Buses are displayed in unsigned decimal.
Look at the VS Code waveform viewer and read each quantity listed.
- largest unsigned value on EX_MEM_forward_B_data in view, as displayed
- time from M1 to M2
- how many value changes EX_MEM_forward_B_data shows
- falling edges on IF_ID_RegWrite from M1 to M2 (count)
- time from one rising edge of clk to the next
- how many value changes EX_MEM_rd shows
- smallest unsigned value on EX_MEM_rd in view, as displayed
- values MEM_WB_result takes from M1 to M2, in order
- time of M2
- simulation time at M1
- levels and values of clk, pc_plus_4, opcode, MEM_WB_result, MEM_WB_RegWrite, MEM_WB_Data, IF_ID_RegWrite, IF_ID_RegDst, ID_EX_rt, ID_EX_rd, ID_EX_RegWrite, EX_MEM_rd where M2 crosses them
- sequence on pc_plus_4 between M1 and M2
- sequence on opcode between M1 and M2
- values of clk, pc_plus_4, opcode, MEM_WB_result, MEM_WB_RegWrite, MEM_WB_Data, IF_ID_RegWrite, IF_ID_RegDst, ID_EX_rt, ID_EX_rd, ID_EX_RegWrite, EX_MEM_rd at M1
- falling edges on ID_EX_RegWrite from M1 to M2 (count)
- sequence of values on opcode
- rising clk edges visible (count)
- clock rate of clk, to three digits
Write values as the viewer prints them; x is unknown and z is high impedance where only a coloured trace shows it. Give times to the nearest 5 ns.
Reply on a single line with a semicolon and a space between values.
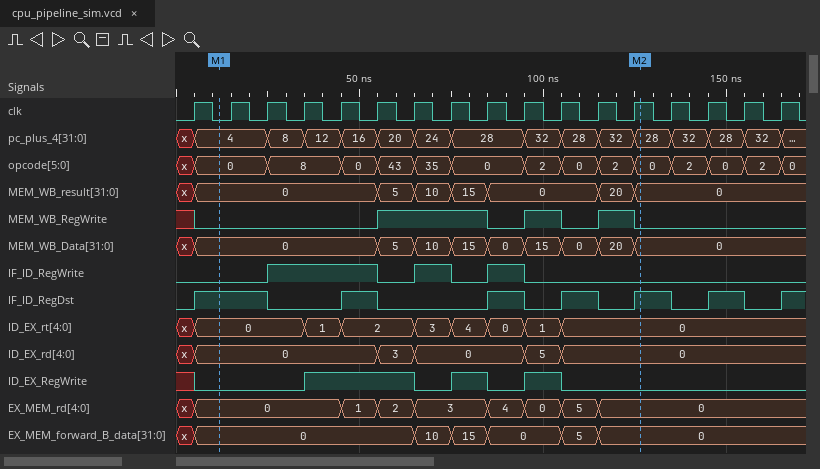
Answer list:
15; 115 ns; 6; 3; 10 ns; 8; 0; 0, 5, 10, 15, 0, 20, 0; 125 ns; 10 ns; clk=1, pc_plus_4=28, opcode=0, MEM_WB_result=0, MEM_WB_RegWrite=0, MEM_WB_Data=0, IF_ID_RegWrite=0, IF_ID_RegDst=1, ID_EX_rt=0, ID_EX_rd=0, ID_EX_RegWrite=0, EX_MEM_rd=0; 4, 8, 12, 16, 20, 24, 28, 32, 28, 32, 28; 0, 8, 0, 43, 35, 0, 2, 0, 2, 0; clk=0, pc_plus_4=4, opcode=0, MEM_WB_result=0, MEM_WB_RegWrite=0, MEM_WB_Data=0, IF_ID_RegWrite=0, IF_ID_RegDst=1, ID_EX_rt=0, ID_EX_rd=0, ID_EX_RegWrite=0, EX_MEM_rd=0; 3; x, 0, 8, 0, 43, 35, 0, 2, 0, 2, 0, 2, 0, 2, 0; 17; 100 MHz
